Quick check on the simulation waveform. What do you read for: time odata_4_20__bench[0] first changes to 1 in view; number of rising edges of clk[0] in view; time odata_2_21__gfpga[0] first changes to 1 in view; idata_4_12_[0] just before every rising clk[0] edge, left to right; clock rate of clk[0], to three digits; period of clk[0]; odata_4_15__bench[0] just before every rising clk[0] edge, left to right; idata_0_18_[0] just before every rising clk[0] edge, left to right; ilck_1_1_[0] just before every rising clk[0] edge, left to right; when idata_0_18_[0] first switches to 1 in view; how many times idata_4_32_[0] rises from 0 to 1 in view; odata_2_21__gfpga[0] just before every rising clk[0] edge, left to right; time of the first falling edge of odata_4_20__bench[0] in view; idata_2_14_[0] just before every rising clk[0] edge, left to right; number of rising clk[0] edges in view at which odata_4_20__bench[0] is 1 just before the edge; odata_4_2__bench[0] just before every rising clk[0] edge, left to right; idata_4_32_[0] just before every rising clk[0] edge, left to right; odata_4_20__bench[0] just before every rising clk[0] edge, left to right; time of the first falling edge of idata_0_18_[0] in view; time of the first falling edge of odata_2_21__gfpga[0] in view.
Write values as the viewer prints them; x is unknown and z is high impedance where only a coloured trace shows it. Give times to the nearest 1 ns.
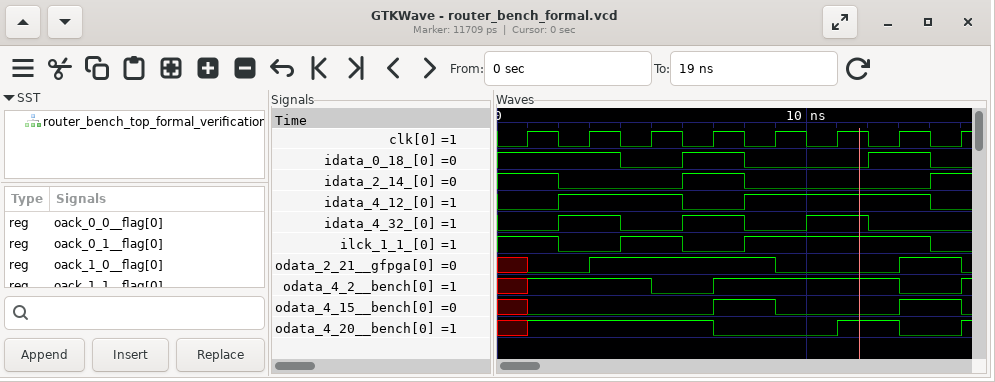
1 ns
8
3 ns
0 1 1 0 1 1 1 0
500 MHz
2 ns
x 0 0 0 1 0 0 1
1 1 0 1 0 0 1 0
1 0 1 0 1 1 1 0
6 ns
3
x 0 1 1 1 0 0 1
7 ns
1 0 0 1 0 0 0 1
4
x 1 1 0 1 1 1 0
0 1 0 1 0 1 0 0
x 1 1 1 0 0 1 0
4 ns
9 ns
